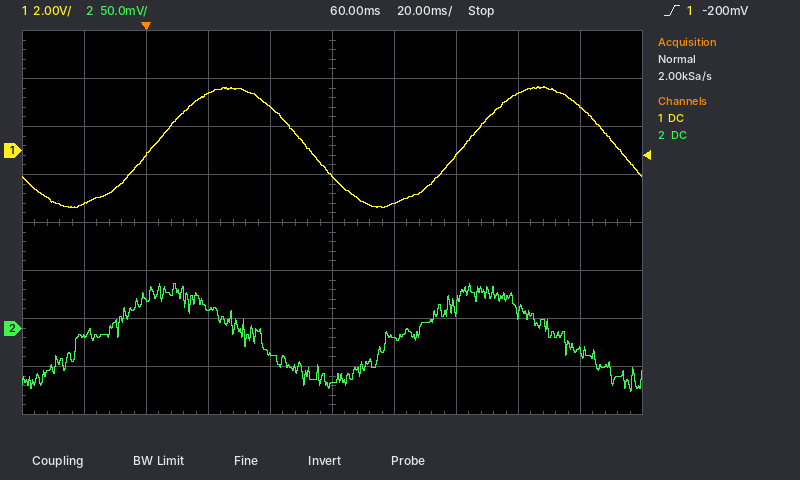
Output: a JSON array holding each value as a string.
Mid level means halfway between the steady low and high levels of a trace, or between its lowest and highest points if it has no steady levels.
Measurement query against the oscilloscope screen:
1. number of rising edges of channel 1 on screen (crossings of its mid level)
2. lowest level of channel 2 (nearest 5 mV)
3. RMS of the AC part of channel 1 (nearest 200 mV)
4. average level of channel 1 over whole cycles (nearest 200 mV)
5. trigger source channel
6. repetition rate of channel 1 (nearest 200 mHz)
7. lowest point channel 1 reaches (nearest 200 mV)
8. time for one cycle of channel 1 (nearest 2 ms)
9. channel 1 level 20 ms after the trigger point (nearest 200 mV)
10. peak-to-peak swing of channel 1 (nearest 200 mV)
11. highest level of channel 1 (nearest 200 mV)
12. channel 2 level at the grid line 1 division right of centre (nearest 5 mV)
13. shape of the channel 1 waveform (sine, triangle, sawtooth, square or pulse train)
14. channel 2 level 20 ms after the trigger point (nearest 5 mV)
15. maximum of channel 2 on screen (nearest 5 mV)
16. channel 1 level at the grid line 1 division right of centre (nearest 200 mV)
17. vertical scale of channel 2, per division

["2", "-65 mV", "1.8 V", "200 mV", "channel 1", "10.0 Hz", "-2.4 V", "100 ms", "2.4 V", "5.0 V", "2.6 V", "-10 mV", "sine", "20 mV", "45 mV", "-2.2 V", "50 mV"]
